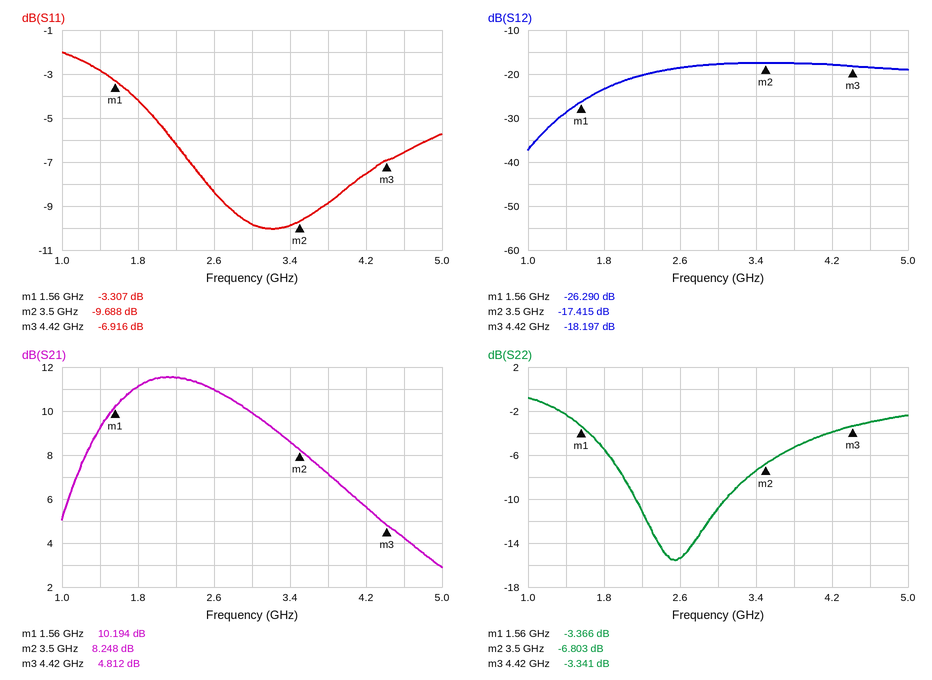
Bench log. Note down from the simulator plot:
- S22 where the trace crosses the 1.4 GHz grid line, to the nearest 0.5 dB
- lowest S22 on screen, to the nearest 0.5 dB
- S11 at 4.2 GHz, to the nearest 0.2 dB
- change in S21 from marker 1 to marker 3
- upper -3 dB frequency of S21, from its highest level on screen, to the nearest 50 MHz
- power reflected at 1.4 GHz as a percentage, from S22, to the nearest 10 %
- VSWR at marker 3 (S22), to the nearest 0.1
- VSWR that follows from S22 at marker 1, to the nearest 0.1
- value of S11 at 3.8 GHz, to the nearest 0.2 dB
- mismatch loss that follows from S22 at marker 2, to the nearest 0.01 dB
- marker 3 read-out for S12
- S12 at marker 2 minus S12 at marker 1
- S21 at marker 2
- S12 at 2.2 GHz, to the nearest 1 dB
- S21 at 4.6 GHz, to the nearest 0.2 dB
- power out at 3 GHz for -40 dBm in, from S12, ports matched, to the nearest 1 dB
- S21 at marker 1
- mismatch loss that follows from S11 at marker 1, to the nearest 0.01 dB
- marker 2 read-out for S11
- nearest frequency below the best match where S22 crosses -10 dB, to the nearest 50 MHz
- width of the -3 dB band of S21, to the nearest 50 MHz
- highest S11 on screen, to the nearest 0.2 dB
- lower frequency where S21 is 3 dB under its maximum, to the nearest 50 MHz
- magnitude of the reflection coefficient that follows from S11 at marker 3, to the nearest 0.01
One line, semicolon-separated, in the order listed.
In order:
-2.5 dB; -15.5 dB; -7.6 dB; -5.382 dB; 3.40 GHz; 60 %; 5.3; 5.2; -8.8 dB; 1.02 dB; -18.197 dB; 8.875 dB; 8.248 dB; -20 dB; 4.2 dB; -58 dBm; 10.194 dB; 2.73 dB; -9.688 dB; 2.15 GHz; 2.10 GHz; -2.0 dB; 1.30 GHz; 0.45
